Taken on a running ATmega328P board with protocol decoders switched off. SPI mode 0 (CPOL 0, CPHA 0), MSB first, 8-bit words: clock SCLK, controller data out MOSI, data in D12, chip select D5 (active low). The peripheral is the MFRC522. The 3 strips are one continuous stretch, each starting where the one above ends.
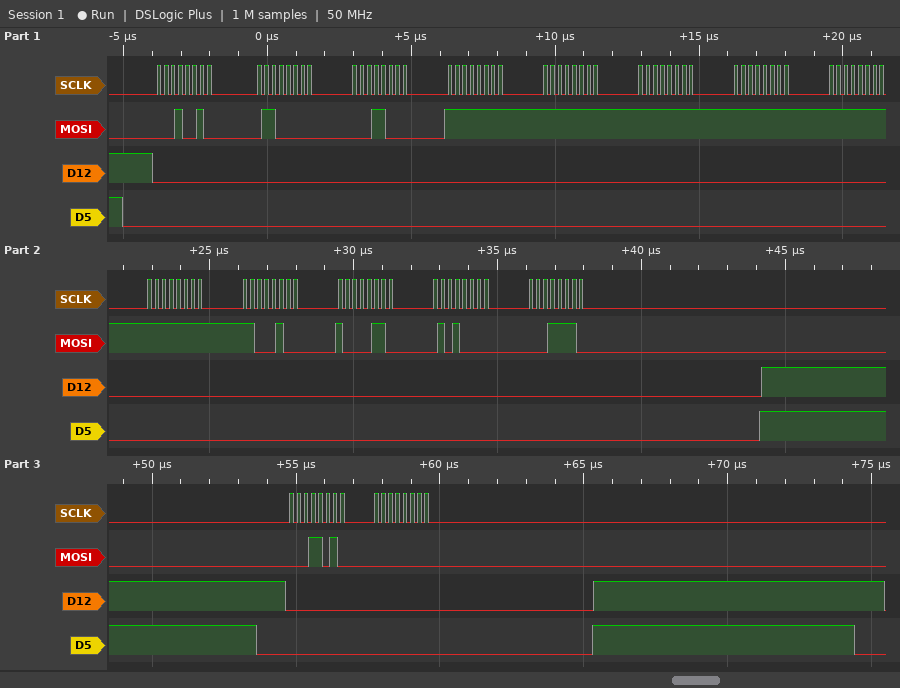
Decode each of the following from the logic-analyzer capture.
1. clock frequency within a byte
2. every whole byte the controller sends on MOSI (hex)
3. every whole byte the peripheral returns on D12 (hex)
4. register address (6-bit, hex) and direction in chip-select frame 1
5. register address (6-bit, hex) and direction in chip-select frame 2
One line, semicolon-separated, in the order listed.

4 MHz; 12 60 18 FF FF FF FF FF FF C4 86 50 1E 1A 00; 00 00 00 00 00 00 00 00 00 00 00 00 00 00 00; 0x09 write; 0x0D write
